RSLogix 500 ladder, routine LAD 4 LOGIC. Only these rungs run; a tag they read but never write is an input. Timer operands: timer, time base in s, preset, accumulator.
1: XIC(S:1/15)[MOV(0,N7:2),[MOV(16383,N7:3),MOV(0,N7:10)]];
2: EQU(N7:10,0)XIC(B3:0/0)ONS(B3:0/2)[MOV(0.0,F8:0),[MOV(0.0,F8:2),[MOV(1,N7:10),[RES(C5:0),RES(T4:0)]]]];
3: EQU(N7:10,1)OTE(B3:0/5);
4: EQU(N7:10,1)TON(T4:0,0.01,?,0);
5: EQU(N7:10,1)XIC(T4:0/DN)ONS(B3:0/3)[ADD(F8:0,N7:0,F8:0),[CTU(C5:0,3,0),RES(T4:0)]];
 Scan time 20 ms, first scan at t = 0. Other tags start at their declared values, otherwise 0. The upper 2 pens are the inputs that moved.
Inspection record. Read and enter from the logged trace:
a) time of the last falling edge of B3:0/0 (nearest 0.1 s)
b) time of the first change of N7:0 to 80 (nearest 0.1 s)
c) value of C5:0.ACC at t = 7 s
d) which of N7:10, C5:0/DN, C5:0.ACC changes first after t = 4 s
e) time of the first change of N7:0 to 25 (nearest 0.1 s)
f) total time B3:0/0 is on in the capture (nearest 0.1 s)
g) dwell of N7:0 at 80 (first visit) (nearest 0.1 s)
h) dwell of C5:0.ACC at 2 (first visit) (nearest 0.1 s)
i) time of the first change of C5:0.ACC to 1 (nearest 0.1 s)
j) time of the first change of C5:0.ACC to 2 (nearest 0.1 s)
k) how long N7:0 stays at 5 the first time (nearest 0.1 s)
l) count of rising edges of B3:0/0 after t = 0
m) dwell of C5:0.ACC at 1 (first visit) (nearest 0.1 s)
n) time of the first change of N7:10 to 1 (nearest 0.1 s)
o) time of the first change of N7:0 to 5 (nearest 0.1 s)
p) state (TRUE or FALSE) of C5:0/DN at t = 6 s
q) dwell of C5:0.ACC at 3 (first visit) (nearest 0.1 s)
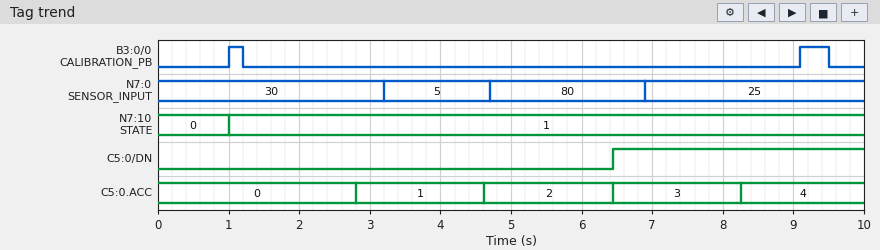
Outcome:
9.5 s
4.7 s
3
C5:0.ACC
6.9 s
0.6 s
2.2 s
1.8 s
2.8 s
4.6 s
1.5 s
2
1.8 s
1.0 s
3.2 s
FALSE
1.8 s
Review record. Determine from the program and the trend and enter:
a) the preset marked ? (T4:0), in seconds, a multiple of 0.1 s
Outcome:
1.8 s
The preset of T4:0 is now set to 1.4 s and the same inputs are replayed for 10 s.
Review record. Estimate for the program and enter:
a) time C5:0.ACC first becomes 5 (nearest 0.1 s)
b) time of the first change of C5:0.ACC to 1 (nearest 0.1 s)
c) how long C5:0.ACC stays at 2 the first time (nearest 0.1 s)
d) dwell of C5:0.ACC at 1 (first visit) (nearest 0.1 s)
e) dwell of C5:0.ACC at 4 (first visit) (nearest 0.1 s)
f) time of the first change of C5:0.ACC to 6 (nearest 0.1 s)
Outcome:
8.1 s
2.4 s
1.4 s
1.4 s
1.4 s
9.5 s
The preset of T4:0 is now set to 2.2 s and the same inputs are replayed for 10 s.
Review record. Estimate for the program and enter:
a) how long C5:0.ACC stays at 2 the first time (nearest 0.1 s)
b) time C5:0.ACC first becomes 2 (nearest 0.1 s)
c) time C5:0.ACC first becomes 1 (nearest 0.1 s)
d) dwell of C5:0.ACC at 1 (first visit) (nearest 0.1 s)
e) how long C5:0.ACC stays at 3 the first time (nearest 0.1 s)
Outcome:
2.2 s
5.4 s
3.2 s
2.2 s
2.2 s
